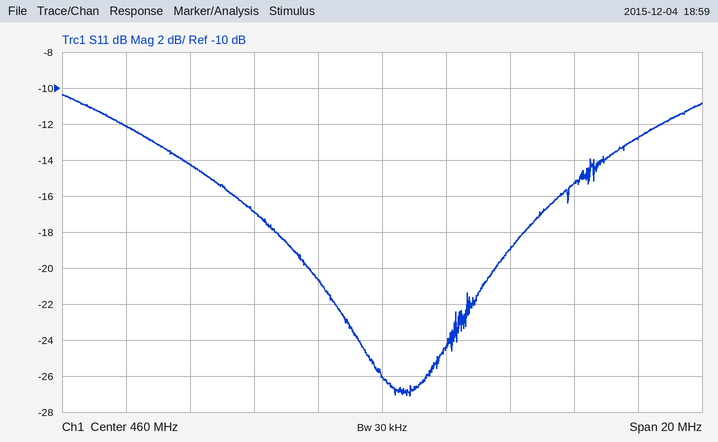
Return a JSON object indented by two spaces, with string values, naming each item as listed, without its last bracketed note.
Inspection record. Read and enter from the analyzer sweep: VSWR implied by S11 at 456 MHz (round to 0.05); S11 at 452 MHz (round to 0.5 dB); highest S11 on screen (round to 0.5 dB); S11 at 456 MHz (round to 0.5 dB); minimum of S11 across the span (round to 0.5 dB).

{
  "VSWR implied by S11 at 456 MHz": "1.35",
  "S11 at 452 MHz": "-12.0 dB",
  "highest S11 on screen": "-10.5 dB",
  "S11 at 456 MHz": "-17.0 dB",
  "minimum of S11 across the span": "-27.0 dB"
}
